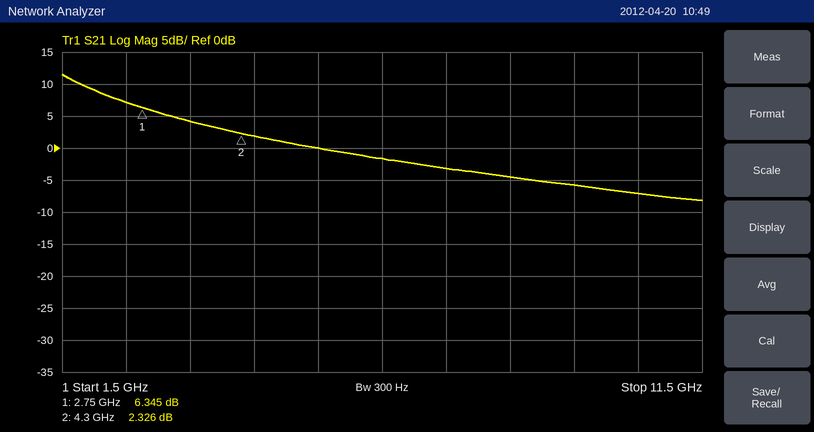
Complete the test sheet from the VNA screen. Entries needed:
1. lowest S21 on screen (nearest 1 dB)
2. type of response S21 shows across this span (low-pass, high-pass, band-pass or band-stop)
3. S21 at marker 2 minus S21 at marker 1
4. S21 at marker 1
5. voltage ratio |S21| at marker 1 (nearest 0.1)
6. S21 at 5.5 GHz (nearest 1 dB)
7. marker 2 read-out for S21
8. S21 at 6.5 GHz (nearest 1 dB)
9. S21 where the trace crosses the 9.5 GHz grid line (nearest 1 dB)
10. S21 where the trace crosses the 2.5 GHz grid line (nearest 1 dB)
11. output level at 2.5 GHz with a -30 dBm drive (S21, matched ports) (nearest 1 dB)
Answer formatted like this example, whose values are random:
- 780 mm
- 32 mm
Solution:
- -8 dB
- low-pass
- -4.019 dB
- 6.345 dB
- 2.1
- 0 dB
- 2.326 dB
- -2 dB
- -6 dB
- 7 dB
- -23 dBm
